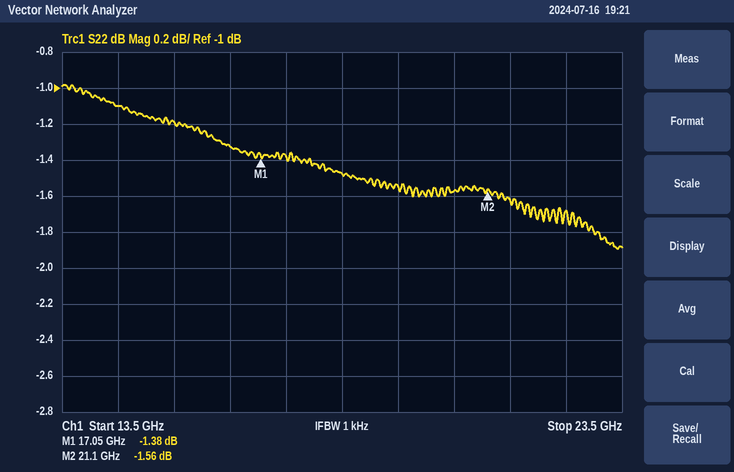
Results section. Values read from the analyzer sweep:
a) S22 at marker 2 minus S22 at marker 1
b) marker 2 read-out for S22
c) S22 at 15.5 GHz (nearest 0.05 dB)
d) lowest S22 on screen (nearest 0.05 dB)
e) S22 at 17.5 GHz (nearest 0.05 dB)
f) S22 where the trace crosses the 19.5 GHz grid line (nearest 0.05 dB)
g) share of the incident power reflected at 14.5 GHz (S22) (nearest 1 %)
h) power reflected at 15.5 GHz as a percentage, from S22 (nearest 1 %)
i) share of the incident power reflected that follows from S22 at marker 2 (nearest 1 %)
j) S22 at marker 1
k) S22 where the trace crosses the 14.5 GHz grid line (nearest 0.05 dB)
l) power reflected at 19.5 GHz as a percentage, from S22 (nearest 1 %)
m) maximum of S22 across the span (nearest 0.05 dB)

-0.18 dB
-1.56 dB
-1.20 dB
-1.90 dB
-1.40 dB
-1.55 dB
78 %
76 %
70 %
-1.38 dB
-1.10 dB
70 %
-1.00 dB
